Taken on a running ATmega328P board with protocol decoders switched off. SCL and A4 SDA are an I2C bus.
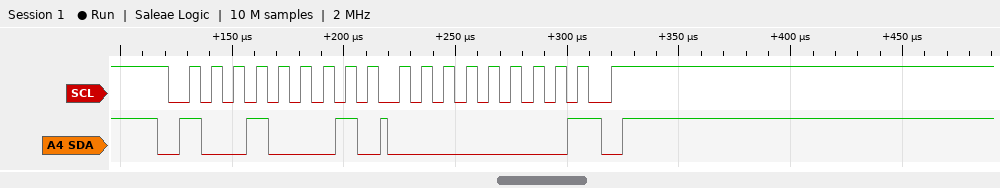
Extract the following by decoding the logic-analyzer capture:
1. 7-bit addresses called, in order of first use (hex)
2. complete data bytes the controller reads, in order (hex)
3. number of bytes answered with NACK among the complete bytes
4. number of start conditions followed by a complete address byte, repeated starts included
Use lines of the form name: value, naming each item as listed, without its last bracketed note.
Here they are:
7-bit addresses called, in order of first use: 0x48
complete data bytes the controller reads, in order: 00
number of bytes answered with NACK among the complete bytes: 1
number of start conditions followed by a complete address byte, repeated starts included: 1
